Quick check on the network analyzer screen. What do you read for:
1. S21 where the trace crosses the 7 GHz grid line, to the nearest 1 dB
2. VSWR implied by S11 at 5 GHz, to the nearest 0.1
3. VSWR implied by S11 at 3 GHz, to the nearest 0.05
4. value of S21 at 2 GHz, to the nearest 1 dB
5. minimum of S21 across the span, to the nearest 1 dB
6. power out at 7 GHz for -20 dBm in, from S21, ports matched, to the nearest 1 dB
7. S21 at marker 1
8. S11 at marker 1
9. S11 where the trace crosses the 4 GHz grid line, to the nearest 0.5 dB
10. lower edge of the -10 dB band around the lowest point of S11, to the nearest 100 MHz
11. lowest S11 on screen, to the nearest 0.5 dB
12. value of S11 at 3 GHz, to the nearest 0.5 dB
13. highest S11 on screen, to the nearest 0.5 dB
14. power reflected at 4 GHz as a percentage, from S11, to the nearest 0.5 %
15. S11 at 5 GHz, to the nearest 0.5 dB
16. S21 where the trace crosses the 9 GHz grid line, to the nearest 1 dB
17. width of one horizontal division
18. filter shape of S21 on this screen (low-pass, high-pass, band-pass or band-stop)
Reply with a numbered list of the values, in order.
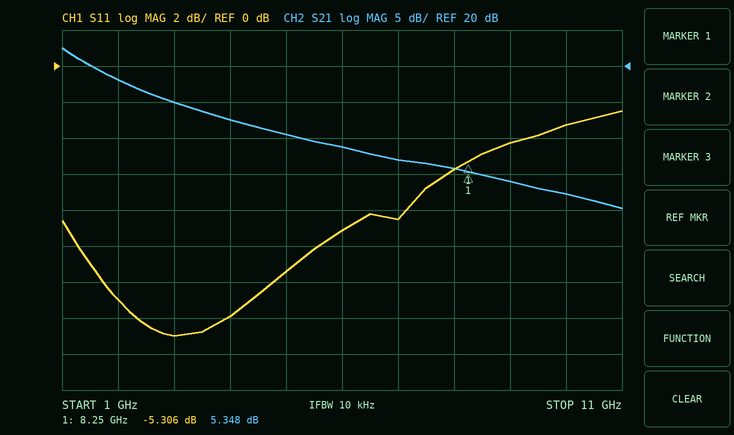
1. 7 dB
2. 1.7
3. 1.45
4. 18 dB
5. 0 dB
6. -13 dBm
7. 5.348 dB
8. -5.306 dB
9. -14.0 dB
10. 1.3 GHz
11. -15.0 dB
12. -15.0 dB
13. -2.5 dB
14. 4.0 %
15. -11.5 dB
16. 4 dB
17. 1 GHz
18. low-pass
